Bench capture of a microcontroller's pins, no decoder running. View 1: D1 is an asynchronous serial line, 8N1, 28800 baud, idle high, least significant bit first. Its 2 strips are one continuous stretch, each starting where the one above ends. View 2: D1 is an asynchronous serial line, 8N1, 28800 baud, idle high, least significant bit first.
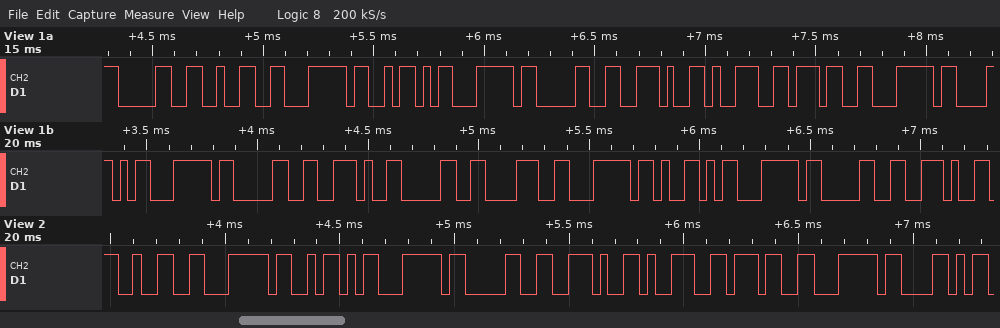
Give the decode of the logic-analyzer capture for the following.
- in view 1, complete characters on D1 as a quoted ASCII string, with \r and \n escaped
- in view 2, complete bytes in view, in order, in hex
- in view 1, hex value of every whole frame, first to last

"02|Z|0.97|X|0.08|Y|0."
32 7C 5A 7C 30 2E 39 37 7C 58
0x30 0x32 0x7C 0x5A 0x7C 0x30 0x2E 0x39 0x37 0x7C 0x58 0x7C 0x30 0x2E 0x30 0x38 0x7C 0x59 0x7C 0x30 0x2E
